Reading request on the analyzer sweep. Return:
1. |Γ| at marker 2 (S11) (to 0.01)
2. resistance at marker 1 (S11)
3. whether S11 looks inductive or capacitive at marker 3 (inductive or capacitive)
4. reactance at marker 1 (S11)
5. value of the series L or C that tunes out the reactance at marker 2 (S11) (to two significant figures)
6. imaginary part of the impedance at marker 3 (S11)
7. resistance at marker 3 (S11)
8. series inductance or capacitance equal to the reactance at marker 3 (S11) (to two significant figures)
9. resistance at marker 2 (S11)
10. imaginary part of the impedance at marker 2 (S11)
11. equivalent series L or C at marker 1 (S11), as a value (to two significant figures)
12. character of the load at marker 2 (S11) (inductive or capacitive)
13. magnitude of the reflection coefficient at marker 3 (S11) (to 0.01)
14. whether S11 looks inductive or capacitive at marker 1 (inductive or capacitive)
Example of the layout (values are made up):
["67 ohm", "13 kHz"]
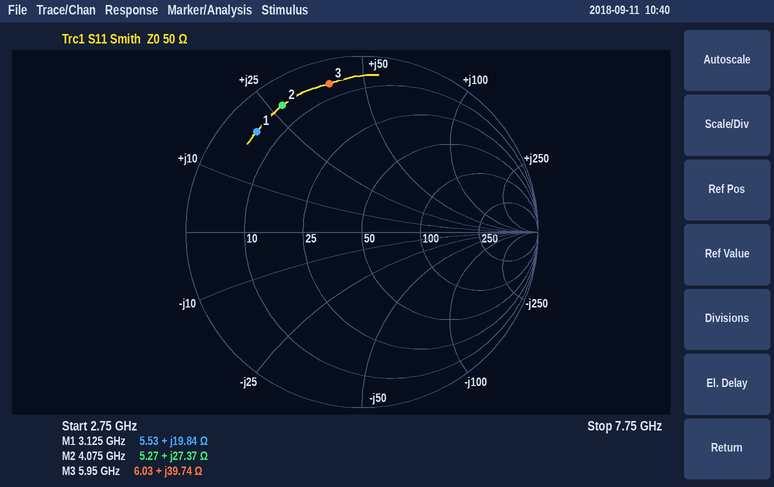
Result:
["0.85", "5.53 Ω", "inductive", "+19.84 Ω", "1.4 pF", "+39.74 Ω", "6.03 Ω", "1.1 nH", "5.27 Ω", "+27.37 Ω", "1.0 nH", "inductive", "0.86", "inductive"]
